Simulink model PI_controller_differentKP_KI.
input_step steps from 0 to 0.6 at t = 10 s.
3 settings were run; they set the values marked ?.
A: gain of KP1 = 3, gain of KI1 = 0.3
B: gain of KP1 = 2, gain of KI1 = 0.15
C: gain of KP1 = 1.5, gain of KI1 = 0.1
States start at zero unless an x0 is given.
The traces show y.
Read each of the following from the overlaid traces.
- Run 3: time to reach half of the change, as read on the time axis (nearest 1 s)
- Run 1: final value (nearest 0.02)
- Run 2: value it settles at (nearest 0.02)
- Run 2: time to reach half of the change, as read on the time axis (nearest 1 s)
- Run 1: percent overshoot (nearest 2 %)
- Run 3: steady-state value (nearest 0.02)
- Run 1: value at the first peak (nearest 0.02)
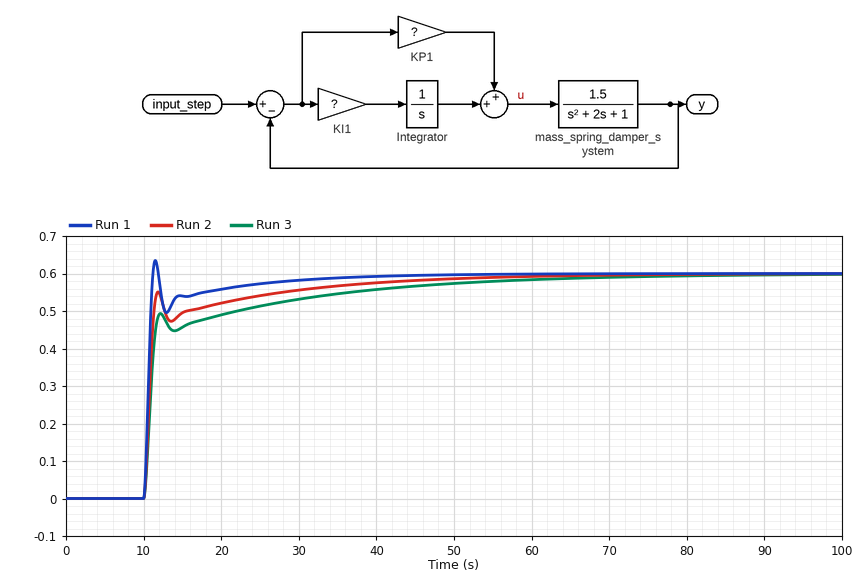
11 s
0.60
0.60
11 s
6 %
0.60
0.64
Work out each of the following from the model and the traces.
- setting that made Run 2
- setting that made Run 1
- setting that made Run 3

B
A
C
